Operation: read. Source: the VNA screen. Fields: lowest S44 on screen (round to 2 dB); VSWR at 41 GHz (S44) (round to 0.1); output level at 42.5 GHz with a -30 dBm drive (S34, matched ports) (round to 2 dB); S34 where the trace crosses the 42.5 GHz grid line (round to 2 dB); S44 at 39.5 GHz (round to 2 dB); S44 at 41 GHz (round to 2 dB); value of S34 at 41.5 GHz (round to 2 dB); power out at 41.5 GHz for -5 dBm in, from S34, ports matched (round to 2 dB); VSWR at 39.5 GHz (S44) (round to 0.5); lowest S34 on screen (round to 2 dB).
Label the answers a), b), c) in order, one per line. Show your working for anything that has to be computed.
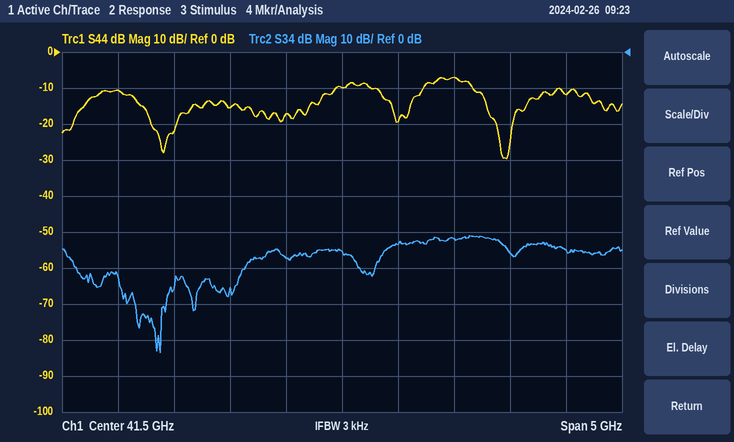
a) -30 dB
b) |Γ| = 10^(-18/20) = 0.1259; VSWR = (1 + 0.1259)/(1 − 0.1259) ≈ 1.3
c) -30 dBm + (-52 dB) = -82 dBm
d) -52 dB
e) -10 dB
f) -18 dB
g) -56 dB
h) -5 dBm + (-56 dB) = -60 dBm
i) |Γ| = 10^(-10/20) = 0.3162; VSWR = (1 + 0.3162)/(1 − 0.3162) ≈ 1.92, so 2.0 to the nearest 0.5
j) -84 dB
